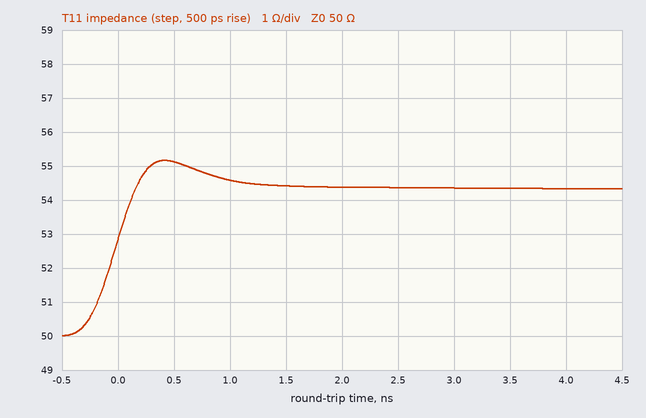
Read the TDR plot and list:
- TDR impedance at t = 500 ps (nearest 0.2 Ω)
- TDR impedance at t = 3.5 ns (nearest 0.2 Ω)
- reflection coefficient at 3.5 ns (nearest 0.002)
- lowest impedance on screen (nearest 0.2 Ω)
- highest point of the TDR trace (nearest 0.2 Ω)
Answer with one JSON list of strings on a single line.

["55.2 Ω", "54.4 Ω", "+0.042", "50.0 Ω", "55.2 Ω"]
